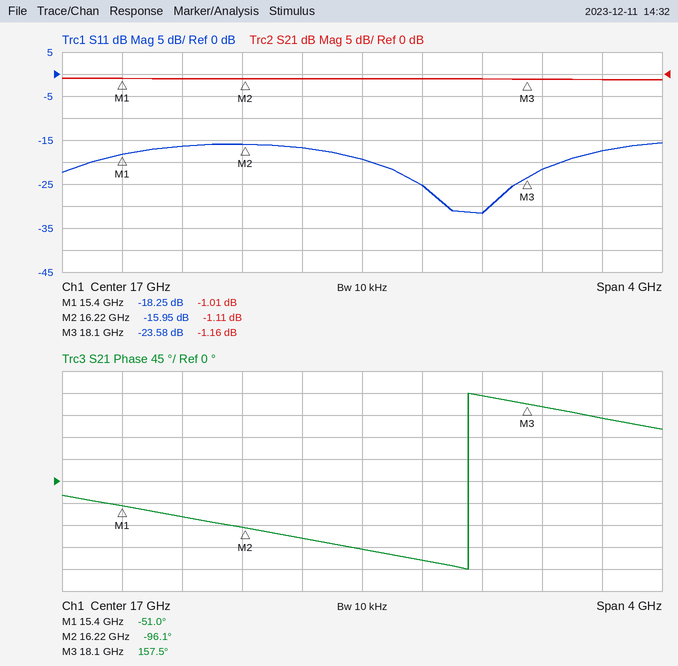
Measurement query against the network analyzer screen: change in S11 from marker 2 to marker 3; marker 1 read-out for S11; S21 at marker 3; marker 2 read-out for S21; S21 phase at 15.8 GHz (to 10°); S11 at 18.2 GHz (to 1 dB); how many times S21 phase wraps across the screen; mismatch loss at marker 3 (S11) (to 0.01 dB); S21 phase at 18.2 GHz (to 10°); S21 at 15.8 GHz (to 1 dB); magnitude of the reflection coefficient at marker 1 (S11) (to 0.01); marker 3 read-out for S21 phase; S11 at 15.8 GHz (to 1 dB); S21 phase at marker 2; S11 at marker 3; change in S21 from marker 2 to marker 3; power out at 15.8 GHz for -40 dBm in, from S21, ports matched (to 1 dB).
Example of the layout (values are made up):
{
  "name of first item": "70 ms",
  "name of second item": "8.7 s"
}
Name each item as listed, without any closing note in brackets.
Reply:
{
  "change in S11 from marker 2 to marker 3": "-7.63 dB",
  "marker 1 read-out for S11": "-18.25 dB",
  "S21 at marker 3": "-1.16 dB",
  "marker 2 read-out for S21": "-1.11 dB",
  "S21 phase at 15.8 GHz": "-70°",
  "S11 at 18.2 GHz": "-22 dB",
  "how many times S21 phase wraps across the screen": "1",
  "mismatch loss at marker 3 (S11)": "0.02 dB",
  "S21 phase at 18.2 GHz": "150°",
  "S21 at 15.8 GHz": "-1 dB",
  "magnitude of the reflection coefficient at marker 1 (S11)": "0.12",
  "marker 3 read-out for S21 phase": "157.5°",
  "S11 at 15.8 GHz": "-16 dB",
  "S21 phase at marker 2": "-96.1°",
  "S11 at marker 3": "-23.58 dB",
  "change in S21 from marker 2 to marker 3": "-0.05 dB",
  "power out at 15.8 GHz for -40 dBm in, from S21, ports matched": "-41 dBm"
}
